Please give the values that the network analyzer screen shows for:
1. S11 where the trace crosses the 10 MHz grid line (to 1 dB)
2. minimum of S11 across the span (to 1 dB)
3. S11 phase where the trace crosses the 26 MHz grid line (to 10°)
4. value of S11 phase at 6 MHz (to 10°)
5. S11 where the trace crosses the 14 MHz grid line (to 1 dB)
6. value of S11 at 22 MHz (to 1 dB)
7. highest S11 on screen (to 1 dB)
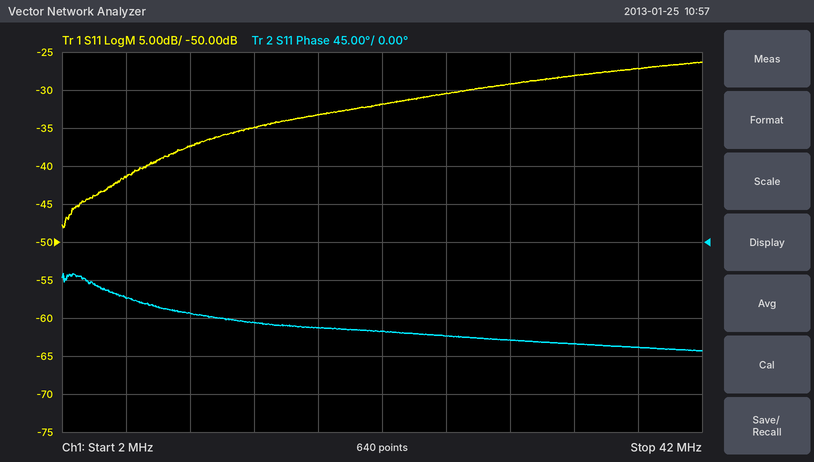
-37 dB
-48 dB
-110°
-70°
-35 dB
-32 dB
-26 dB
